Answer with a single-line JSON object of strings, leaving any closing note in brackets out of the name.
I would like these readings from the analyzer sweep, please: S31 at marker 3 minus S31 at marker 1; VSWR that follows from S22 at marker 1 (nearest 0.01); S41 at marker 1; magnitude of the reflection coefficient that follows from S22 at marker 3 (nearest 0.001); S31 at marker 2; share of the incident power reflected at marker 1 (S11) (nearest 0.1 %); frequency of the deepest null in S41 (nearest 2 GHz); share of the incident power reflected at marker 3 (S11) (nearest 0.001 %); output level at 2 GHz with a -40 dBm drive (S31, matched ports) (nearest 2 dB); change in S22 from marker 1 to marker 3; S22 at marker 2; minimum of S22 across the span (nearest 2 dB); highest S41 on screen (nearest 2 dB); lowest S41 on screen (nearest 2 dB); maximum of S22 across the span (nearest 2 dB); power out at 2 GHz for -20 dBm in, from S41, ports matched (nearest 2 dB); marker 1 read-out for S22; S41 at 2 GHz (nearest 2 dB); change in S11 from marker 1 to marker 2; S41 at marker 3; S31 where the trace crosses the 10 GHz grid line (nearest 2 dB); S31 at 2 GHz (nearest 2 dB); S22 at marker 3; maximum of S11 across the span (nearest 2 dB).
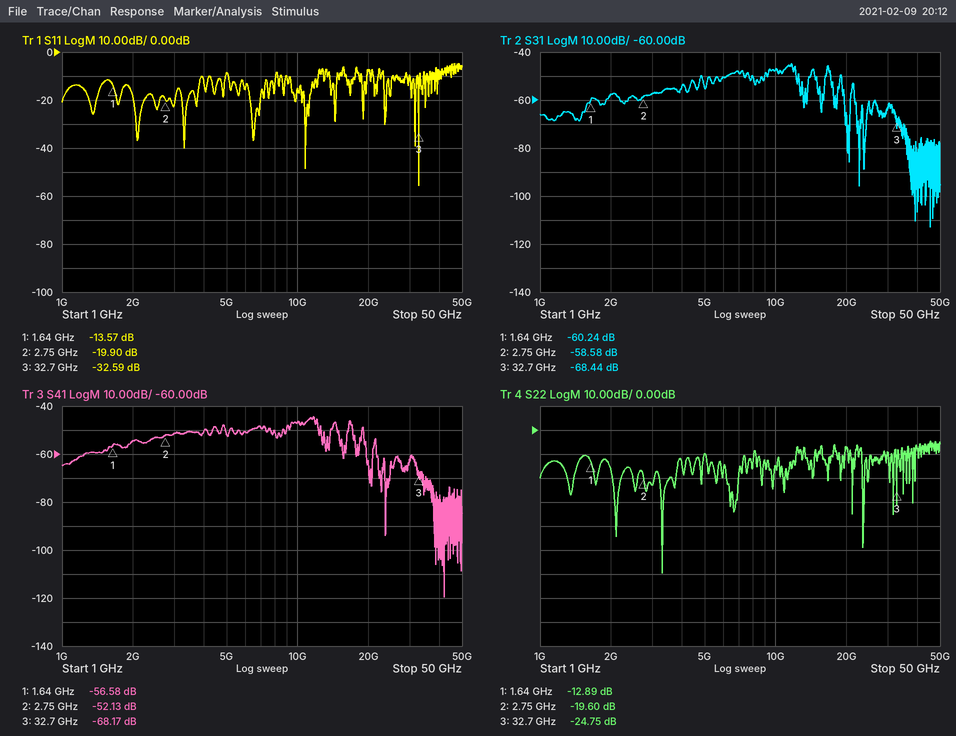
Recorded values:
{"S31 at marker 3 minus S31 at marker 1": "-8.20 dB", "VSWR that follows from S22 at marker 1": "1.59", "S41 at marker 1": "-56.58 dB", "magnitude of the reflection coefficient that follows from S22 at marker 3": "0.058", "S31 at marker 2": "-58.58 dB", "share of the incident power reflected at marker 1 (S11)": "4.4 %", "frequency of the deepest null in S41": "42 GHz", "share of the incident power reflected at marker 3 (S11)": "0.055 %", "output level at 2 GHz with a -40 dBm drive (S31, matched ports)": "-98 dBm", "change in S22 from marker 1 to marker 3": "-11.86 dB", "S22 at marker 2": "-19.60 dB", "minimum of S22 across the span": "-60 dB", "highest S41 on screen": "-44 dB", "lowest S41 on screen": "-120 dB", "maximum of S22 across the span": "-4 dB", "power out at 2 GHz for -20 dBm in, from S41, ports matched": "-74 dBm", "marker 1 read-out for S22": "-12.89 dB", "S41 at 2 GHz": "-54 dB", "change in S11 from marker 1 to marker 2": "-6.33 dB", "S41 at marker 3": "-68.17 dB", "S31 where the trace crosses the 10 GHz grid line": "-48 dB", "S31 at 2 GHz": "-58 dB", "S22 at marker 3": "-24.75 dB", "maximum of S11 across the span": "-4 dB"}
